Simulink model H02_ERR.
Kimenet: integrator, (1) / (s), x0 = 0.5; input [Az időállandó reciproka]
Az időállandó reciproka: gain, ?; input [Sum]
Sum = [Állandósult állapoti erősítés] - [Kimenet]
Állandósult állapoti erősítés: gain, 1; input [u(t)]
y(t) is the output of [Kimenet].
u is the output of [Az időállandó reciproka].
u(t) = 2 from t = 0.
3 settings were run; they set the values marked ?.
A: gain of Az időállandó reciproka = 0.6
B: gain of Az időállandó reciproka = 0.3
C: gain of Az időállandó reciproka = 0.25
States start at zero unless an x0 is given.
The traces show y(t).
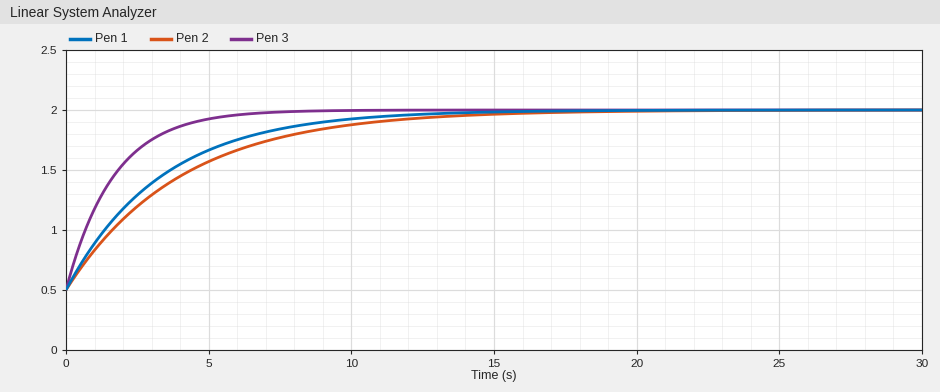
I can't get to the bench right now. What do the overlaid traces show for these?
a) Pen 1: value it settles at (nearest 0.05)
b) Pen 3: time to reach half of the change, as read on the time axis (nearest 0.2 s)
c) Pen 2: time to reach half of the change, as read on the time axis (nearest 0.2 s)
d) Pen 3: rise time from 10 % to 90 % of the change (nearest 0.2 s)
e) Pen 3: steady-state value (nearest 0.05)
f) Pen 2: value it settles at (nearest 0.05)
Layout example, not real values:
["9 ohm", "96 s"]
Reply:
["2.00", "1.2 s", "2.8 s", "3.6 s", "2.00", "2.00"]
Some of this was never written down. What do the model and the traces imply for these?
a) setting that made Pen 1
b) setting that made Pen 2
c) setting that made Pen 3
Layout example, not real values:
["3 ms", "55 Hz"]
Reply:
["B", "C", "A"]
